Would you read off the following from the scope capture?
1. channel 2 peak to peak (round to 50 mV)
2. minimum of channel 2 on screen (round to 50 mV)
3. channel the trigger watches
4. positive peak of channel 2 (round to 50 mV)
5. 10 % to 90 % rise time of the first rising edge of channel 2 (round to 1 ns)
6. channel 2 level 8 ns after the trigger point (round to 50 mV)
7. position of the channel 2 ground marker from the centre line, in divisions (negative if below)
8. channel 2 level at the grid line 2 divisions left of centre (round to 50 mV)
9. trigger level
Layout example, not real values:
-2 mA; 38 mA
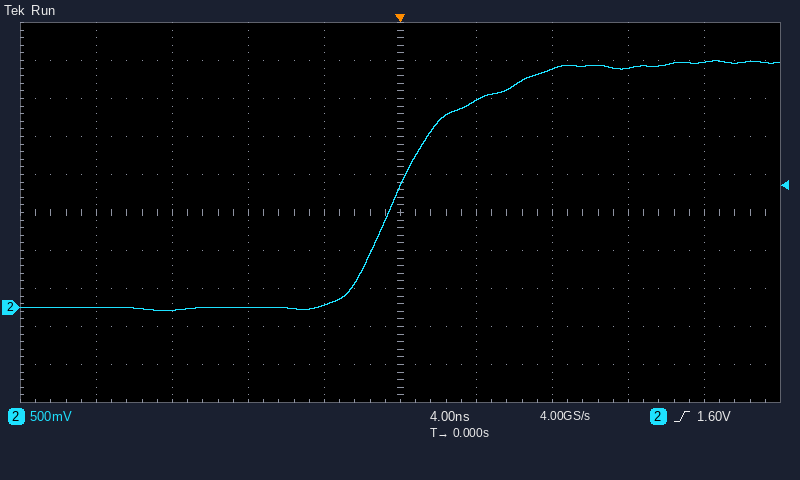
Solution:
3.30 V; -50 mV; channel 2; 3.25 V; 8 ns; 3.15 V; -2.5 div; 0 mV; 1.60 V
